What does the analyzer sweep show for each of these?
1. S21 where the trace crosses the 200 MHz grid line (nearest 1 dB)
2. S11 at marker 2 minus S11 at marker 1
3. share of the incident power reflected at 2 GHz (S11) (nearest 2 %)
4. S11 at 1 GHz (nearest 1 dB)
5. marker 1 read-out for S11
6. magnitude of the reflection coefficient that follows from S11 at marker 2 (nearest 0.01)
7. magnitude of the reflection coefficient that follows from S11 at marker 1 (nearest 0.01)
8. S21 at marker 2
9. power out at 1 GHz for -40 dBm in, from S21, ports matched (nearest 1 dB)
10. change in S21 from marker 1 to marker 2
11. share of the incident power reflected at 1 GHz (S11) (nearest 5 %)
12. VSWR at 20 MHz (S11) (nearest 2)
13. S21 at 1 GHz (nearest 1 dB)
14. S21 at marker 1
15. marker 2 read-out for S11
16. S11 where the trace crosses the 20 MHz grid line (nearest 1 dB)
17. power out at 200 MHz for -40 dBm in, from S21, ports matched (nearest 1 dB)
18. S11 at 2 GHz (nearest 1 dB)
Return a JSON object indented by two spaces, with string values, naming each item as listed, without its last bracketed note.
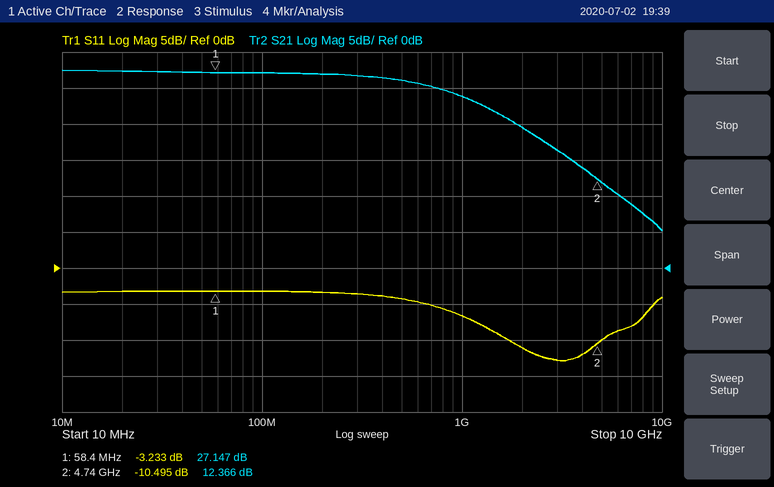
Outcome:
{
  "S21 where the trace crosses the 200 MHz grid line": "27 dB",
  "S11 at marker 2 minus S11 at marker 1": "-7.262 dB",
  "share of the incident power reflected at 2 GHz (S11)": "8 %",
  "S11 at 1 GHz": "-7 dB",
  "marker 1 read-out for S11": "-3.233 dB",
  "magnitude of the reflection coefficient that follows from S11 at marker 2": "0.30",
  "magnitude of the reflection coefficient that follows from S11 at marker 1": "0.69",
  "S21 at marker 2": "12.366 dB",
  "power out at 1 GHz for -40 dBm in, from S21, ports matched": "-16 dBm",
  "change in S21 from marker 1 to marker 2": "-14.781 dB",
  "share of the incident power reflected at 1 GHz (S11)": "20 %",
  "VSWR at 20 MHz (S11)": "6",
  "S21 at 1 GHz": "24 dB",
  "S21 at marker 1": "27.147 dB",
  "marker 2 read-out for S11": "-10.495 dB",
  "S11 where the trace crosses the 20 MHz grid line": "-3 dB",
  "power out at 200 MHz for -40 dBm in, from S21, ports matched": "-13 dBm",
  "S11 at 2 GHz": "-11 dB"
}
